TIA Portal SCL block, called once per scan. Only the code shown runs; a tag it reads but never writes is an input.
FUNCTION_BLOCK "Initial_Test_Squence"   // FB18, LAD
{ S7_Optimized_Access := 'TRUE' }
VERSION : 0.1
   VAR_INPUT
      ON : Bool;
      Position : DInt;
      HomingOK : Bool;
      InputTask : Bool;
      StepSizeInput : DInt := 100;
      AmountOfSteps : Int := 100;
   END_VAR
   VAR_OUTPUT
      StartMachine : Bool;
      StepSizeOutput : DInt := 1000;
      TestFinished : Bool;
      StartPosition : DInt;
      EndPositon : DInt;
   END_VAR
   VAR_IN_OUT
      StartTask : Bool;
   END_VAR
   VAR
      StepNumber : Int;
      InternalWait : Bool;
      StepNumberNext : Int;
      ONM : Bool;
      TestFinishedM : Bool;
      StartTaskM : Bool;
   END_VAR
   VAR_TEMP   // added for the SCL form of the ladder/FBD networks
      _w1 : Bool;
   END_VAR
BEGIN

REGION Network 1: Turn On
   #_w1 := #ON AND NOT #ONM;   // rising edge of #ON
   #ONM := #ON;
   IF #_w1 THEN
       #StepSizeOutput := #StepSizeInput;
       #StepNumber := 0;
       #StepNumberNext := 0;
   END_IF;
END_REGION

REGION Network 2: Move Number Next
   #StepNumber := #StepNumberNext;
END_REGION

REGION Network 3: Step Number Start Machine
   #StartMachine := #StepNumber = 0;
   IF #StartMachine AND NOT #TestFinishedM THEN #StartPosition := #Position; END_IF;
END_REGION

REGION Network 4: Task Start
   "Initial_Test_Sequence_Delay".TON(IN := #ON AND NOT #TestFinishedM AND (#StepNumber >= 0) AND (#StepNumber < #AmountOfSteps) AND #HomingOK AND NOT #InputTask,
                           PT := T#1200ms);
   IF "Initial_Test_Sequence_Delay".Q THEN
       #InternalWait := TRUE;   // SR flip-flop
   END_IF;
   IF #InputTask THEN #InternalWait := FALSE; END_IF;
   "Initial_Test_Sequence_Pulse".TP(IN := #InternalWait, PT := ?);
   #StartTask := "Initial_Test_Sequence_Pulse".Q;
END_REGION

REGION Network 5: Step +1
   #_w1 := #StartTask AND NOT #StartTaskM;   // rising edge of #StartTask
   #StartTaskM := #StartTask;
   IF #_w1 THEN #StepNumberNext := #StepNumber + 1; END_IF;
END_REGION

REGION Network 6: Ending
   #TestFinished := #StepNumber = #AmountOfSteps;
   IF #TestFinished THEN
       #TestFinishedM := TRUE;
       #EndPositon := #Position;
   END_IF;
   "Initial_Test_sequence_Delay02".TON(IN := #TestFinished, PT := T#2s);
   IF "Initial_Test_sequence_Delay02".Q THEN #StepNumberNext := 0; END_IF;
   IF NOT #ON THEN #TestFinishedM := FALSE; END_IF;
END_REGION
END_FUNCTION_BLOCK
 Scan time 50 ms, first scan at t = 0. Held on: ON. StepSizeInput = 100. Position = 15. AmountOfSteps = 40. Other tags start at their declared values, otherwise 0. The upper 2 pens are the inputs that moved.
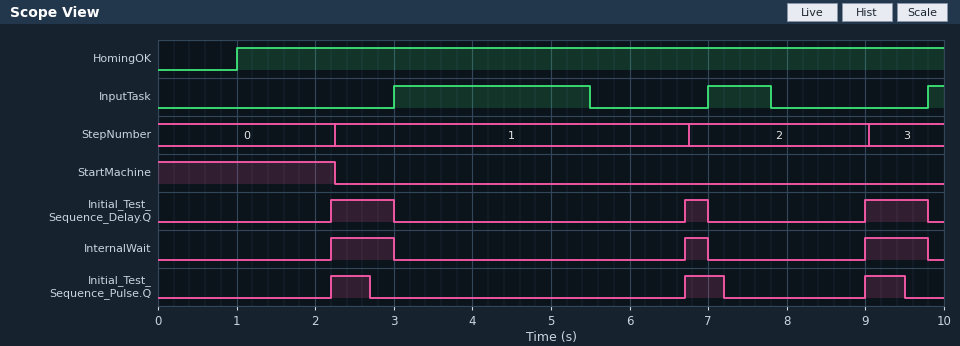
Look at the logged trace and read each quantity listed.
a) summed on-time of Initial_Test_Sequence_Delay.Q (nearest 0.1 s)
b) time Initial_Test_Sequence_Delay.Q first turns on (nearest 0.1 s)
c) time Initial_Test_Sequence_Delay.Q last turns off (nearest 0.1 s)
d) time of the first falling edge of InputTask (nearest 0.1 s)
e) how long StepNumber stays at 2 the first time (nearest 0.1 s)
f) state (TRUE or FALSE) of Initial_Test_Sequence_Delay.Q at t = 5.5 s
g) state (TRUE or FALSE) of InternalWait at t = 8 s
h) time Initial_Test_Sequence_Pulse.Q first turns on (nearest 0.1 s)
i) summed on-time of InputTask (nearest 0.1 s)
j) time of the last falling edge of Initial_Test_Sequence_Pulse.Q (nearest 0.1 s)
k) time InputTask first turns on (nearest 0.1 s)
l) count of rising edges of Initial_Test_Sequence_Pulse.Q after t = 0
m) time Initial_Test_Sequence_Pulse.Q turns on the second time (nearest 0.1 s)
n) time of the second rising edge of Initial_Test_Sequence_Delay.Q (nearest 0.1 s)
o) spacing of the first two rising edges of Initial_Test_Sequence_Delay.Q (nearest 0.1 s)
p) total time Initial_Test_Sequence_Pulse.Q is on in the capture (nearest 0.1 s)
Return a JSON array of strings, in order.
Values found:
["1.9 s", "2.2 s", "9.8 s", "5.5 s", "2.3 s", "FALSE", "FALSE", "2.2 s", "3.5 s", "9.5 s", "3.0 s", "3", "6.7 s", "6.7 s", "4.5 s", "1.5 s"]
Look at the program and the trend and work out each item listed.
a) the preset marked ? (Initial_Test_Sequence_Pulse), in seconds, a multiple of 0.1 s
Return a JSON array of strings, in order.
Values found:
["0.5 s"]
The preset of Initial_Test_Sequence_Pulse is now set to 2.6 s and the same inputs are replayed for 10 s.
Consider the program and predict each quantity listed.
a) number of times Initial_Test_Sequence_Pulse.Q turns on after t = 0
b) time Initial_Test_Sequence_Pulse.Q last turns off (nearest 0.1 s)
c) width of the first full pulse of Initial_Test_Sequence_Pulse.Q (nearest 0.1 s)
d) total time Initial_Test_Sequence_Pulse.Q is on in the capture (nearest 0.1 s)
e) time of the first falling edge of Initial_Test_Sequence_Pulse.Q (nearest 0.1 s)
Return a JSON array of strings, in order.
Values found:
["2", "9.3 s", "2.6 s", "5.2 s", "4.8 s"]
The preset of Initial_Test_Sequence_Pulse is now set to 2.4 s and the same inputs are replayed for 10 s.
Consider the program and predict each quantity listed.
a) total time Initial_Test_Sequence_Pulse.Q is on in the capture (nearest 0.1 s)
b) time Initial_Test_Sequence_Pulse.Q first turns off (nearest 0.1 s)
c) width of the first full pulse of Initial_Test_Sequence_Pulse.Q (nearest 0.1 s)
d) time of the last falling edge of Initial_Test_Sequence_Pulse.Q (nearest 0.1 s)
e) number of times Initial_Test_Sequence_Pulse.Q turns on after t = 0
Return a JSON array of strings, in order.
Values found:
["4.8 s", "4.6 s", "2.4 s", "9.1 s", "2"]
